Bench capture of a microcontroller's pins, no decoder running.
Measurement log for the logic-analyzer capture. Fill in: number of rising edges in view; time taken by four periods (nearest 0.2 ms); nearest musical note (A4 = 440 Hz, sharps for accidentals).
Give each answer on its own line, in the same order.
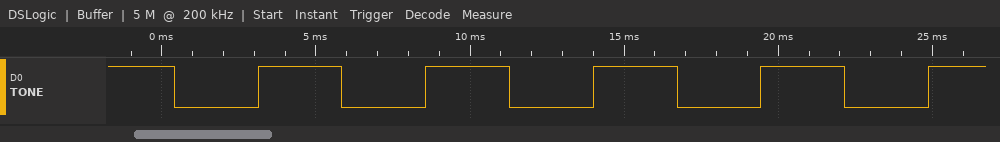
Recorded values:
5
21.8 ms
F#3
